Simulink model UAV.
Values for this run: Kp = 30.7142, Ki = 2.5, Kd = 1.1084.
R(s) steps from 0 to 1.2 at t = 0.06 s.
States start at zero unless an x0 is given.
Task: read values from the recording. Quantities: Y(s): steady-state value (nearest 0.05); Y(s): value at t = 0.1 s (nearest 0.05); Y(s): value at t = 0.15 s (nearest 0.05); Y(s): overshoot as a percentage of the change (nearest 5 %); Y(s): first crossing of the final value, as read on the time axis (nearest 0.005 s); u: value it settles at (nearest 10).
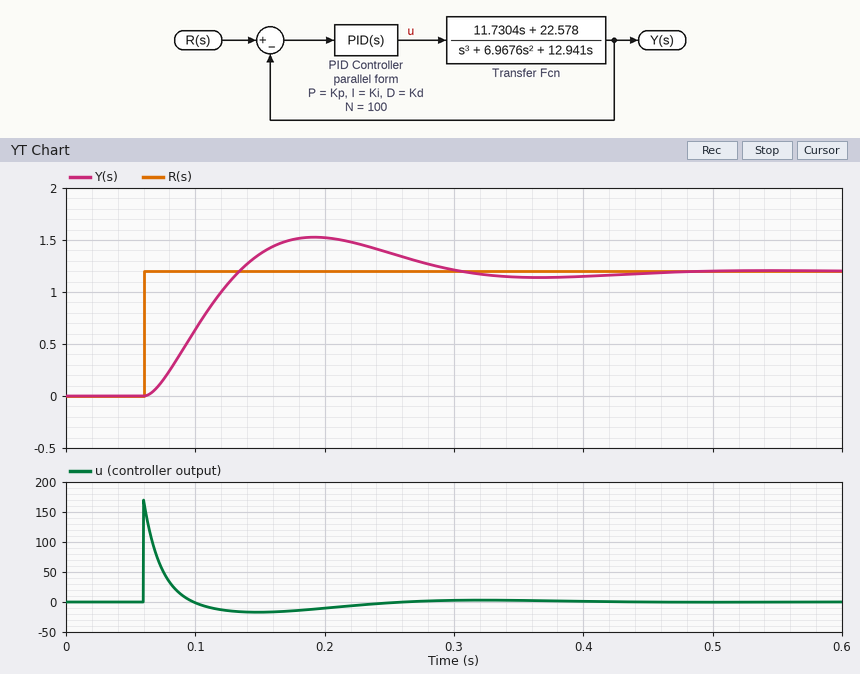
1.20
0.65
1.35
25 %
0.135 s
0
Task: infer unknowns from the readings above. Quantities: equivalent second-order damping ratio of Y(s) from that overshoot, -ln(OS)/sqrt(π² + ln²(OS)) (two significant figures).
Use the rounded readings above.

0.40
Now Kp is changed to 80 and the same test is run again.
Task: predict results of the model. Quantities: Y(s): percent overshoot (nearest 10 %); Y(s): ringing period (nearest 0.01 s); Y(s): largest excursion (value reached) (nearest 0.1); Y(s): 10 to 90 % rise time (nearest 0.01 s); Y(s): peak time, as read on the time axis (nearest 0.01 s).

50 %
0.20 s
1.8
0.03 s
0.15 s
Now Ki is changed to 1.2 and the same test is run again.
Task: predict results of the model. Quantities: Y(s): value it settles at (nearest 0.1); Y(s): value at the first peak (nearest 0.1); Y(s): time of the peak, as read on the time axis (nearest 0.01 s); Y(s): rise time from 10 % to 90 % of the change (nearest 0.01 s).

1.2
1.5
0.19 s
0.05 s
